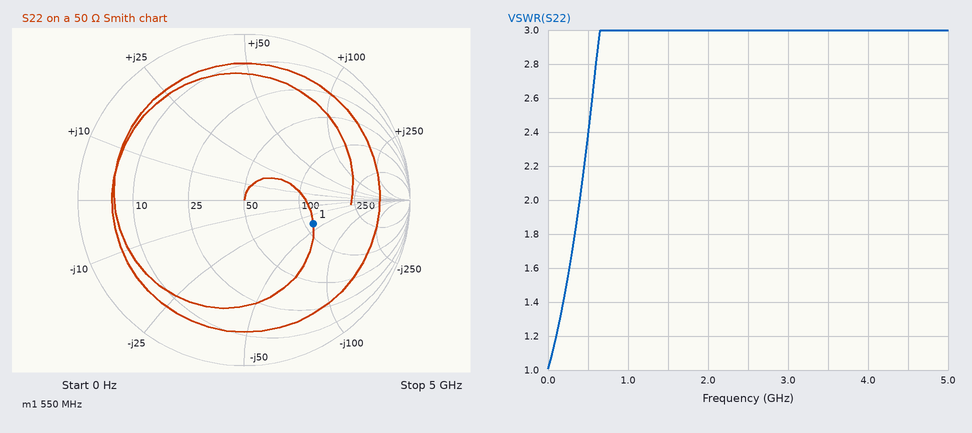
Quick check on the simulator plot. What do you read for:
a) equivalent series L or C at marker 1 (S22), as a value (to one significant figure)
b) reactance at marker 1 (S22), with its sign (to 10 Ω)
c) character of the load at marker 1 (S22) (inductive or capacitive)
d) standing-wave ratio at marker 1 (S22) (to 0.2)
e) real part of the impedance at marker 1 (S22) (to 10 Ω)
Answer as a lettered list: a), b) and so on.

a) 7 pF
b) -40 Ω
c) capacitive
d) 2.6
e) 110 Ω
